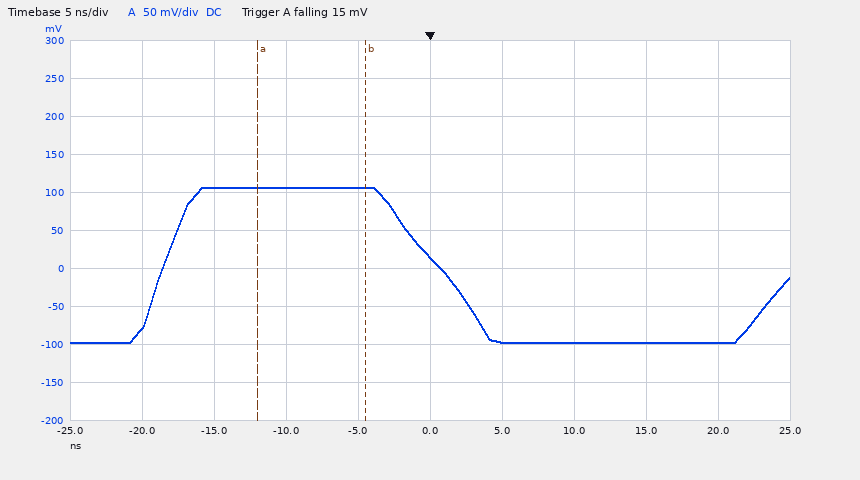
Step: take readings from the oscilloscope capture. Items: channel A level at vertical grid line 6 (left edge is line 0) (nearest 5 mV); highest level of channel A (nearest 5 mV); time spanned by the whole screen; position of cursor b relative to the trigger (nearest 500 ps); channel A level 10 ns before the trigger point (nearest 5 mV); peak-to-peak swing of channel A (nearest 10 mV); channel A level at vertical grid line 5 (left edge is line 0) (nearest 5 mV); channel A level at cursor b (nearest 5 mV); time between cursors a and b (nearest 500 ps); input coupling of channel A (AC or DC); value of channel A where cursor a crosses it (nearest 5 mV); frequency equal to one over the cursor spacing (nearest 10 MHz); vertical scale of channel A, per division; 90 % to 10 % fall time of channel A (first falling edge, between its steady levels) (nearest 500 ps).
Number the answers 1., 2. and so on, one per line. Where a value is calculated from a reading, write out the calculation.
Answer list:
1. -95 mV
2. 105 mV
3. 50 ns
4. -4.5 ns
5. 105 mV
6. 200 mV
7. 15 mV
8. 105 mV
9. 7.5 ns
10. DC
11. 105 mV
12. 1 / 7.5 ns ≈ 130 MHz
13. 50 mV
14. 6.5 ns
